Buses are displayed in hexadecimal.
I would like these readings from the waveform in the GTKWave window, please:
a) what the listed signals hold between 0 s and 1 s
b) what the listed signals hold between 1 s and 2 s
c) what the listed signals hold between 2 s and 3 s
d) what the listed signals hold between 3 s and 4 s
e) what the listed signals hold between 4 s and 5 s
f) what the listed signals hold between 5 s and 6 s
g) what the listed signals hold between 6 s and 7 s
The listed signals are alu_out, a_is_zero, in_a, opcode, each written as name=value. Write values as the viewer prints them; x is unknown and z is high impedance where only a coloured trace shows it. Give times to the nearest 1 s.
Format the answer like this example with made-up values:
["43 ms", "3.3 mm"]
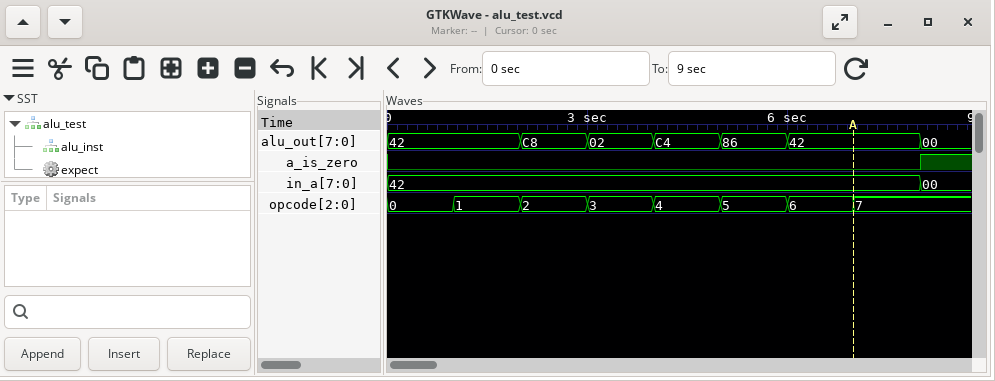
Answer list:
["alu_out=42, a_is_zero=0, in_a=42, opcode=0", "alu_out=42, a_is_zero=0, in_a=42, opcode=1", "alu_out=C8, a_is_zero=0, in_a=42, opcode=2", "alu_out=02, a_is_zero=0, in_a=42, opcode=3", "alu_out=C4, a_is_zero=0, in_a=42, opcode=4", "alu_out=86, a_is_zero=0, in_a=42, opcode=5", "alu_out=42, a_is_zero=0, in_a=42, opcode=6"]
